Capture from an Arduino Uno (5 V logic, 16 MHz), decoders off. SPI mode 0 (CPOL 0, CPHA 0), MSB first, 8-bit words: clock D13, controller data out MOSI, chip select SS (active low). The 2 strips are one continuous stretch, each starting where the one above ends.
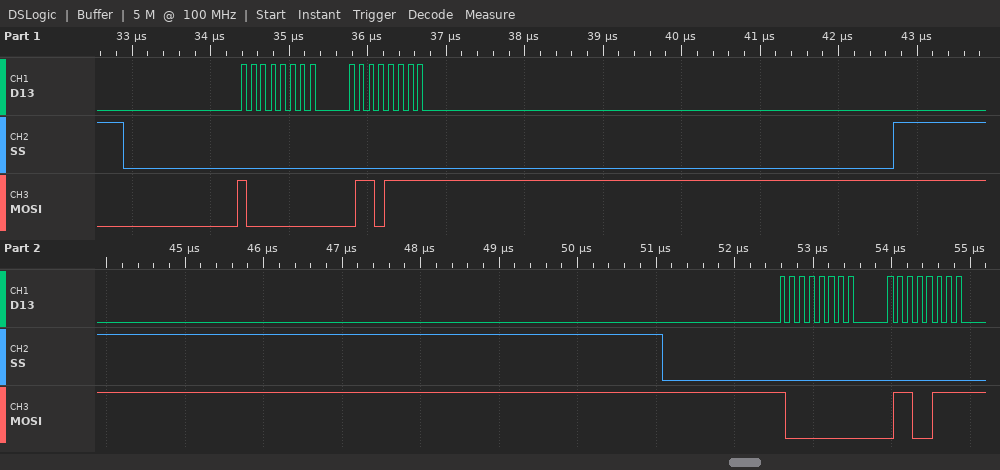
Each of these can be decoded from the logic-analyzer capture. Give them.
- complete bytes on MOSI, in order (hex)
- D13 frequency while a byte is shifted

80 6F 80 67
8 MHz
